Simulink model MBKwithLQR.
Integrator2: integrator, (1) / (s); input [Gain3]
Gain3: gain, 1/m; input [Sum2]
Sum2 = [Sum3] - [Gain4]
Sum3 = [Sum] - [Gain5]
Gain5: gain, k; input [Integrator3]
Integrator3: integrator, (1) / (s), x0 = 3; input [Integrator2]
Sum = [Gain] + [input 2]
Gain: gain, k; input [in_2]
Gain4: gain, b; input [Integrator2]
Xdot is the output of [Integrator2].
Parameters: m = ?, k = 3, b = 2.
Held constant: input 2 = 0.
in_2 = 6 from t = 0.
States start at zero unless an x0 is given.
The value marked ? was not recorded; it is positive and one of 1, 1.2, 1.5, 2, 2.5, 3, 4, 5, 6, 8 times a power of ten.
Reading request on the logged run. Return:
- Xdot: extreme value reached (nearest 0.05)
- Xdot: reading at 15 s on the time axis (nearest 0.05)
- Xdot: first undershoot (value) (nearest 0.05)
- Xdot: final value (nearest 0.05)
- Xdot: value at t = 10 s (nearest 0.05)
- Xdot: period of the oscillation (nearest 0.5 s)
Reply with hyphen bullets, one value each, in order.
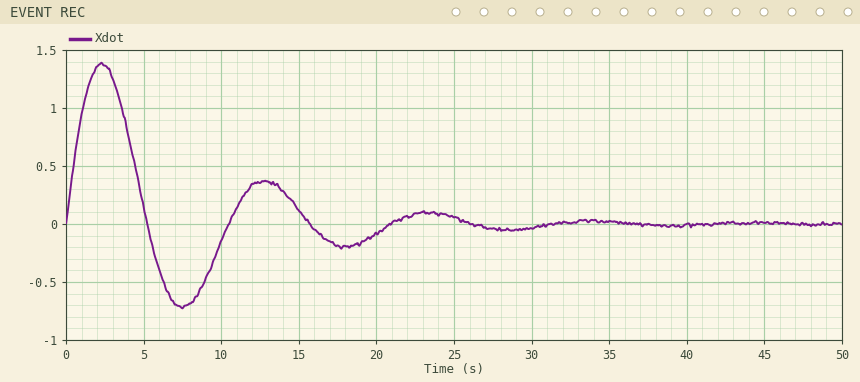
- 1.40
- 0.10
- -0.70
- 0.00
- -0.15
- 10.5 s
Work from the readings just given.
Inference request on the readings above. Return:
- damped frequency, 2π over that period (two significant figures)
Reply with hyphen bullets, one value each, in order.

- 0.60 rad/s
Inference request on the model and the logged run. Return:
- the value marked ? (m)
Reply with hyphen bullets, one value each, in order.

- 8
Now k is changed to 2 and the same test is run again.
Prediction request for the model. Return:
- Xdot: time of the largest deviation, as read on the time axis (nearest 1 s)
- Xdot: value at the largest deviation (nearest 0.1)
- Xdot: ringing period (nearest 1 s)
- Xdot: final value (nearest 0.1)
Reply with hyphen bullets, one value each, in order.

- 3 s
- 1.1
- 13 s
- 0.0
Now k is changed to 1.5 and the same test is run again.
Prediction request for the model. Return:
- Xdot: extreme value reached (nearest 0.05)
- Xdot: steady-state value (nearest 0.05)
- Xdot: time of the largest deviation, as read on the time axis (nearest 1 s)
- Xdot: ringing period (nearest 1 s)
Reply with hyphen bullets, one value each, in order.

- 0.90
- 0.00
- 3 s
- 15 s
